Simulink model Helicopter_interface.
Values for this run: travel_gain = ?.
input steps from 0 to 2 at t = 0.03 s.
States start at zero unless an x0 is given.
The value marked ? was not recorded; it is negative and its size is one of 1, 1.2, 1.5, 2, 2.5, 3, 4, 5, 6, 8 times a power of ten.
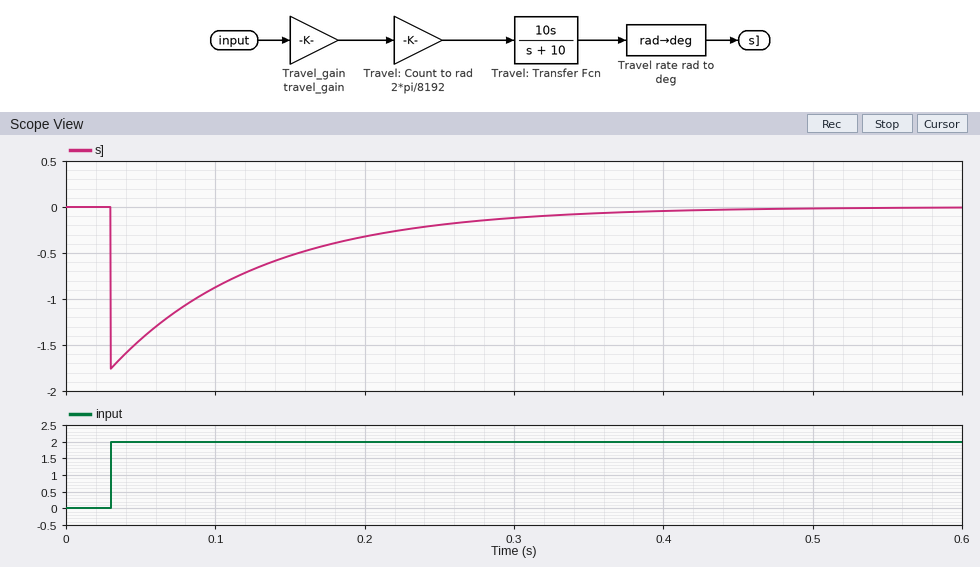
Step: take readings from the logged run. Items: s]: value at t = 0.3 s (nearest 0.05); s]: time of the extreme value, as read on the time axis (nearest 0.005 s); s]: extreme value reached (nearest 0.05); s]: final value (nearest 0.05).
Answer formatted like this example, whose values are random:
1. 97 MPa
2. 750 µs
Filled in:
1. -0.10
2. 0.030 s
3. -1.75
4. 0.00
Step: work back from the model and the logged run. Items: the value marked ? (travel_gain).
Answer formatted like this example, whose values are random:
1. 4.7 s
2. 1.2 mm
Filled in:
1. -2
